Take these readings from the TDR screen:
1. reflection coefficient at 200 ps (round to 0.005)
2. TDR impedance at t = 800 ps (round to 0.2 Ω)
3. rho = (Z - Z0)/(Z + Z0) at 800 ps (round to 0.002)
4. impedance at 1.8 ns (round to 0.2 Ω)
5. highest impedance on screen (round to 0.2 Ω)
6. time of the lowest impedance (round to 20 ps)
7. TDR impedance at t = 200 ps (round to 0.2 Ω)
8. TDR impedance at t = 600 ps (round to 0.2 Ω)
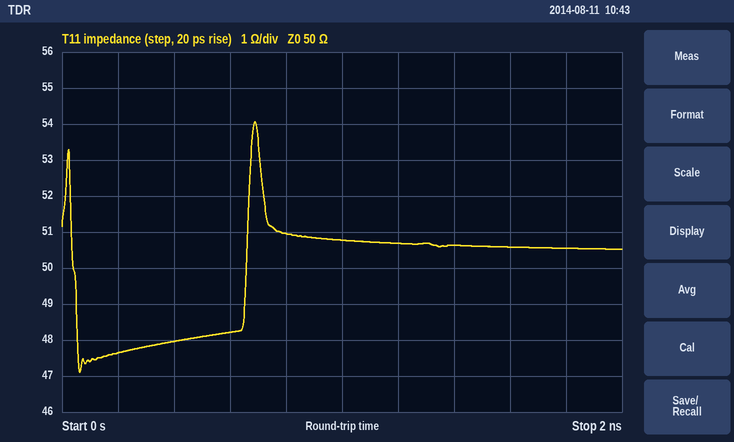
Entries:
-0.025
51.0 Ω
+0.010
50.6 Ω
54.0 Ω
60 ps
47.6 Ω
48.2 Ω
